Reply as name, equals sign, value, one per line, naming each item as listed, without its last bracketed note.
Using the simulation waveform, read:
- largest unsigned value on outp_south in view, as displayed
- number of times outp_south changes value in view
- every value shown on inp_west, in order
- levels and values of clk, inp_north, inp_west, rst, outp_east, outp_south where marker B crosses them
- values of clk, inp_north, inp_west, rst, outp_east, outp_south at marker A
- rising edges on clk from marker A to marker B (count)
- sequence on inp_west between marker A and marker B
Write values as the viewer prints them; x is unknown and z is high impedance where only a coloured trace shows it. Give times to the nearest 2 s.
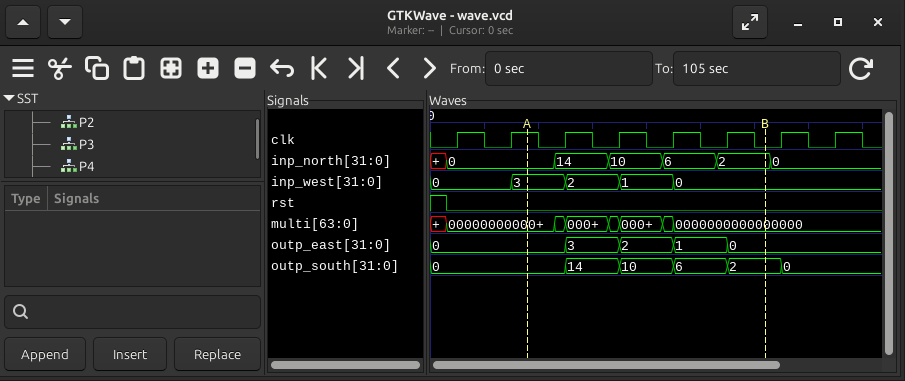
largest unsigned value on outp_south in view, as displayed = 14
number of times outp_south changes value in view = 5
every value shown on inp_west, in order = 0, 3, 2, 1, 0
levels and values of clk, inp_north, inp_west, rst, outp_east, outp_south where marker B crosses them = clk=0, inp_north=2, inp_west=0, rst=0, outp_east=0, outp_south=2
values of clk, inp_north, inp_west, rst, outp_east, outp_south at marker A = clk=1, inp_north=0, inp_west=3, rst=0, outp_east=0, outp_south=0
rising edges on clk from marker A to marker B = 4
sequence on inp_west between marker A and marker B = 3, 2, 1, 0
